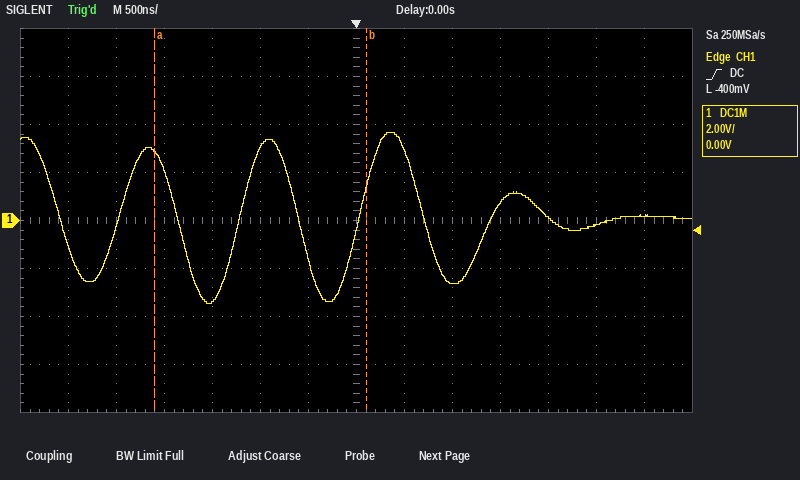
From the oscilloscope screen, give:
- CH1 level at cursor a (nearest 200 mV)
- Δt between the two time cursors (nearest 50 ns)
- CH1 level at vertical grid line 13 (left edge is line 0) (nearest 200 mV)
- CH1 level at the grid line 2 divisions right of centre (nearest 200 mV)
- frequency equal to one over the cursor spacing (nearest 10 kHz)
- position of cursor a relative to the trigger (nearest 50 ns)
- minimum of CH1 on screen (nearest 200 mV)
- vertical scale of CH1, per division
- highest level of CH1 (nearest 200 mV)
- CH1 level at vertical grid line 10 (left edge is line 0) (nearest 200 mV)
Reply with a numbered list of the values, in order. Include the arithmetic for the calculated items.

1. 2.8 V
2. 2.20 µs
3. 200 mV
4. -2.6 V
5. 1 / 2.20 µs ≈ 450 kHz
6. -2.10 µs
7. -3.4 V
8. 2 V
9. 3.6 V
10. 800 mV
